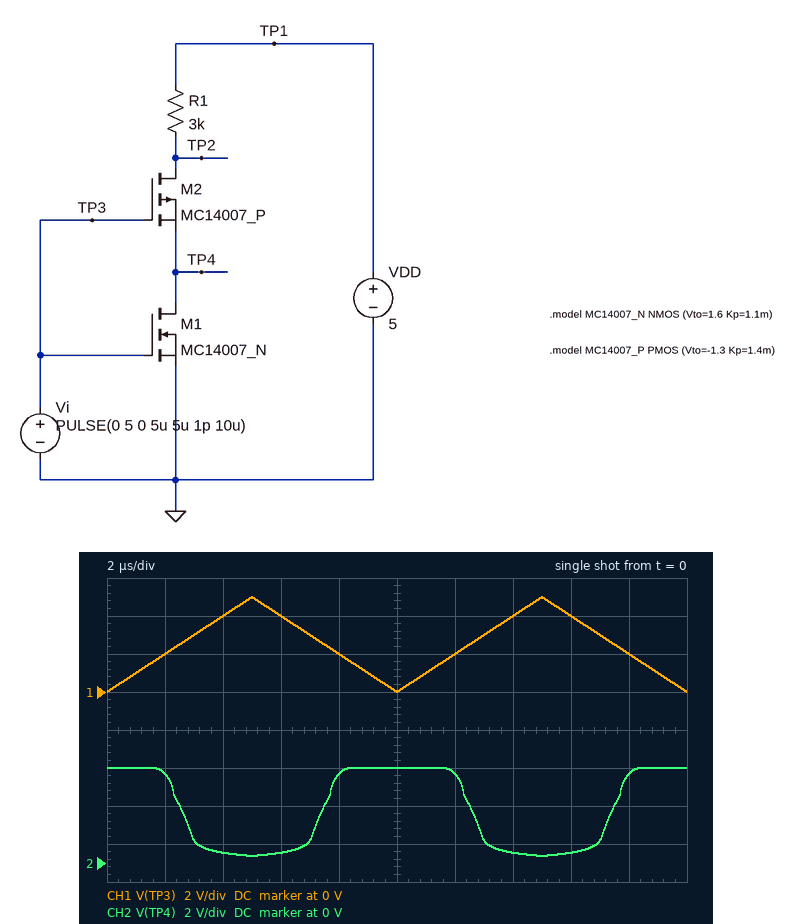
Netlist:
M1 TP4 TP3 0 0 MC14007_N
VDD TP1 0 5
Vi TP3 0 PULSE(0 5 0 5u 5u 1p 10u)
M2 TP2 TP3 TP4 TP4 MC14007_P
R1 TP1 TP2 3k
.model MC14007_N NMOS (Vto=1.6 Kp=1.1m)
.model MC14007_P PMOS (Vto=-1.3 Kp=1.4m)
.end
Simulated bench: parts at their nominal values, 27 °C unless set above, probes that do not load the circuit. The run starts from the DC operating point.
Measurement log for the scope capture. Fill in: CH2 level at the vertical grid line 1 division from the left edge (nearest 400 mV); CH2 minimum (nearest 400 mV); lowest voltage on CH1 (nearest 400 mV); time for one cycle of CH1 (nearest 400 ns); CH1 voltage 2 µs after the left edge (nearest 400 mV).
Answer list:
4.8 V
400 mV
0 V
10.0 µs
2.0 V
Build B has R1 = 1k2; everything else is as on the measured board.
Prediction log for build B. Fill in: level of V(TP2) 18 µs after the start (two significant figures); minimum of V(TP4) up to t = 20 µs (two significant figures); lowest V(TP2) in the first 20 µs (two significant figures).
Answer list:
4.9 V
880 mV
1.6 V
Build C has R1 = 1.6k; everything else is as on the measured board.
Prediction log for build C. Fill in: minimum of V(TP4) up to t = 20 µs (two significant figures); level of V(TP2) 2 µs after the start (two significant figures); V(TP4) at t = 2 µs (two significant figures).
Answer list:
680 mV
4.9 V
4.8 V
